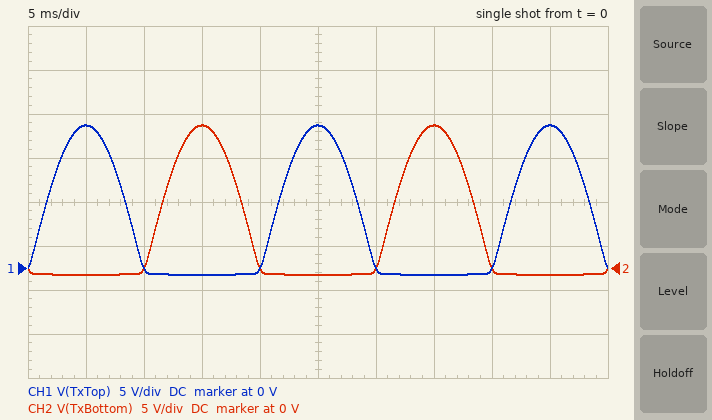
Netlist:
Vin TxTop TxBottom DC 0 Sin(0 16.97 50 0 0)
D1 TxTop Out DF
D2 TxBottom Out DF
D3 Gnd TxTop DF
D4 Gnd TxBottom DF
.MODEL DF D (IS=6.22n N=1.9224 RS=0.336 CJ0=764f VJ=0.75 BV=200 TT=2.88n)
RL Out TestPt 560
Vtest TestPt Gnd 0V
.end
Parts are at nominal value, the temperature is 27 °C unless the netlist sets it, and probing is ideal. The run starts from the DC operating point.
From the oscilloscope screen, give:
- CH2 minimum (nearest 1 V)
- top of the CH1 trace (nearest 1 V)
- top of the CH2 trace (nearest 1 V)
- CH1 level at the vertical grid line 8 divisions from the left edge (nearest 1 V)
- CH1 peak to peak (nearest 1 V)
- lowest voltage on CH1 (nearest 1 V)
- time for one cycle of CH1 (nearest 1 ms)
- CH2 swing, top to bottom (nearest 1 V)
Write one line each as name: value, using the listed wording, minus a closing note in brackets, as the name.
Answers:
CH2 minimum: -1 V
top of the CH1 trace: 16 V
top of the CH2 trace: 16 V
CH1 level at the vertical grid line 8 divisions from the left edge: 0 V
CH1 peak to peak: 17 V
lowest voltage on CH1: -1 V
time for one cycle of CH1: 20 ms
CH2 swing, top to bottom: 17 V
